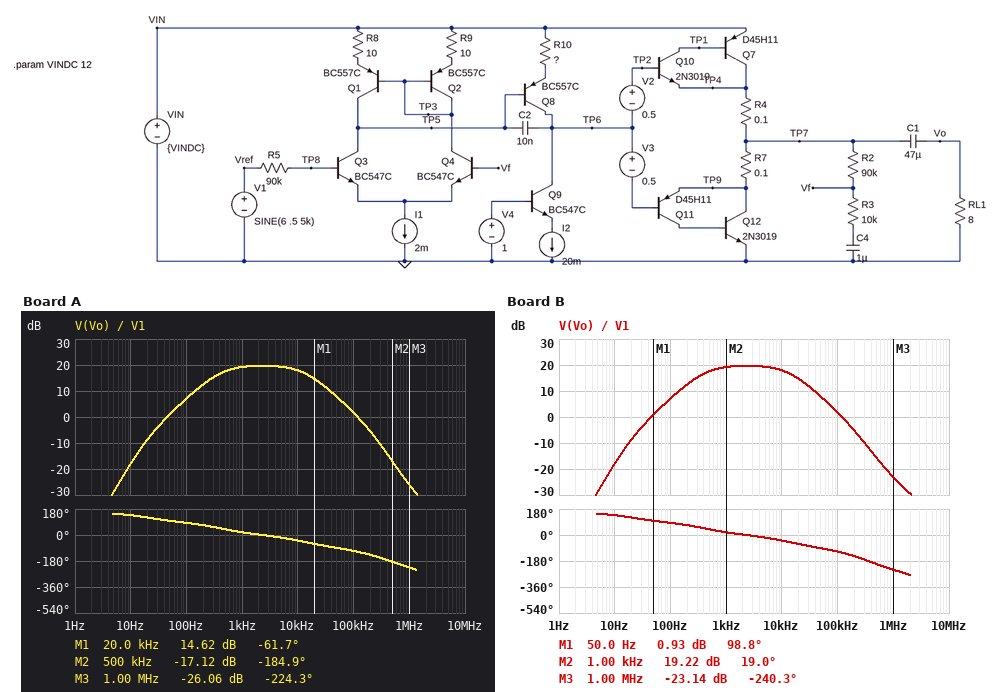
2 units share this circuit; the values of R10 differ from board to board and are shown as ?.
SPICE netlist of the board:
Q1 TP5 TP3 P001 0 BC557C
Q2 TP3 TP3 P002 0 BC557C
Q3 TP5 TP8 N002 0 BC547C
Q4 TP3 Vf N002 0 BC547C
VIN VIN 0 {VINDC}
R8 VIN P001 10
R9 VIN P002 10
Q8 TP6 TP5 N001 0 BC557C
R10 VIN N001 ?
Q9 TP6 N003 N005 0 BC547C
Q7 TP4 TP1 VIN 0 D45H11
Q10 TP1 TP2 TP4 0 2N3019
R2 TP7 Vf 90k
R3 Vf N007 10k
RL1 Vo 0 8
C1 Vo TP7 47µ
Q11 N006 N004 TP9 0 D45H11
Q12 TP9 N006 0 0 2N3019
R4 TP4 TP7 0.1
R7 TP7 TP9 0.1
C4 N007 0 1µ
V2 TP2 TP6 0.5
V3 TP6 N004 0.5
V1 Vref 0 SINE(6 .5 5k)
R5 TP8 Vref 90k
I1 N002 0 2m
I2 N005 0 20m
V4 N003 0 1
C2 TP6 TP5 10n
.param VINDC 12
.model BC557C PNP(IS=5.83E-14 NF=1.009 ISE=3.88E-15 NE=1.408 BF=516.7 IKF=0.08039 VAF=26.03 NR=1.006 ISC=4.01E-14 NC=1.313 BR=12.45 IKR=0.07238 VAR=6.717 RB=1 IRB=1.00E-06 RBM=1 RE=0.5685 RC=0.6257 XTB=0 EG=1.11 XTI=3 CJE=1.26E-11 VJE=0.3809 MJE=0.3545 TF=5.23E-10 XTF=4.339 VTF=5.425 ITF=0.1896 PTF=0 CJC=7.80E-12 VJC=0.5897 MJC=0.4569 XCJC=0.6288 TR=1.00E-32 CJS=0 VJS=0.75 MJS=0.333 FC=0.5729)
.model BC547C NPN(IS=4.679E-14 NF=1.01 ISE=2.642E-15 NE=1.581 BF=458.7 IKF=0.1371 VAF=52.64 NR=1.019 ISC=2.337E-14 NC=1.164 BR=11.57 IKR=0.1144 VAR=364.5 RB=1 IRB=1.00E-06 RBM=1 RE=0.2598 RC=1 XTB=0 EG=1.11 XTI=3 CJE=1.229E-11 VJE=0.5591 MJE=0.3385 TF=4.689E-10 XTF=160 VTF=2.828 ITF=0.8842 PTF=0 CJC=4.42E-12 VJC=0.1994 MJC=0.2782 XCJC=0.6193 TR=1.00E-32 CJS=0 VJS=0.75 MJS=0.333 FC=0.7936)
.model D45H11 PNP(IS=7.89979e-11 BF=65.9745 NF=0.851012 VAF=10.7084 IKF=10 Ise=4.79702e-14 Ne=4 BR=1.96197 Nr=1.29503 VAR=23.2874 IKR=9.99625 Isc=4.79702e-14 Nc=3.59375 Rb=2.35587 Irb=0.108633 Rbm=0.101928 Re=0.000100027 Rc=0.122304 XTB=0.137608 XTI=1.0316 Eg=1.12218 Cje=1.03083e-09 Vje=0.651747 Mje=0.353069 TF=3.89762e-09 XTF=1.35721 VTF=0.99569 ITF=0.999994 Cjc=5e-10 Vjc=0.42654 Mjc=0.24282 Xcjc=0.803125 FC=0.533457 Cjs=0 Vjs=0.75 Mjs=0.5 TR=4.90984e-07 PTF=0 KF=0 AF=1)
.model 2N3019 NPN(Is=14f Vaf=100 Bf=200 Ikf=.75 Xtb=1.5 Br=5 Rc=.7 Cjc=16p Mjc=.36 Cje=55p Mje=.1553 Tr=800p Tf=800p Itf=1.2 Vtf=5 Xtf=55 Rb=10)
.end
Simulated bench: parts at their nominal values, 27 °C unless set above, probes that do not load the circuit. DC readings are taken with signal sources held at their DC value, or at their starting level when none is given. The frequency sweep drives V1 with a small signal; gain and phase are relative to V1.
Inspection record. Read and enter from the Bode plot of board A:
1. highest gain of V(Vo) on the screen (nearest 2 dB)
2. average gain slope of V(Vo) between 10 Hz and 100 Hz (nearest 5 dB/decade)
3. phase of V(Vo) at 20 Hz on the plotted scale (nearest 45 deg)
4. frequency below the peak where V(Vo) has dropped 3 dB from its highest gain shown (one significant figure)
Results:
20 dB
25 dB/decade
135 deg
400 Hz
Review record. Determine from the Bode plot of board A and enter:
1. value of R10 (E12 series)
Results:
15 Ω
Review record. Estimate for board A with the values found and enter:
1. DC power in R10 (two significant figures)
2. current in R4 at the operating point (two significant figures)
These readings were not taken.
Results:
6.0 mW
95 mA
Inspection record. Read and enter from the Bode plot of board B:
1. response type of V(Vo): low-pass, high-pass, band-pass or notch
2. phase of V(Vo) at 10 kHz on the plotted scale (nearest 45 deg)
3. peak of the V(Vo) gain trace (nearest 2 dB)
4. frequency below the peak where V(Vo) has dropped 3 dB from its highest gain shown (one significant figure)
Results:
band-pass
-45 deg
20 dB
400 Hz
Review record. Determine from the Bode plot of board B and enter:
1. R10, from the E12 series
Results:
27 Ω
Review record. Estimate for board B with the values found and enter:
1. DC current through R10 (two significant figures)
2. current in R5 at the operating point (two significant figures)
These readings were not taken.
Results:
20 mA
2.1 µA
